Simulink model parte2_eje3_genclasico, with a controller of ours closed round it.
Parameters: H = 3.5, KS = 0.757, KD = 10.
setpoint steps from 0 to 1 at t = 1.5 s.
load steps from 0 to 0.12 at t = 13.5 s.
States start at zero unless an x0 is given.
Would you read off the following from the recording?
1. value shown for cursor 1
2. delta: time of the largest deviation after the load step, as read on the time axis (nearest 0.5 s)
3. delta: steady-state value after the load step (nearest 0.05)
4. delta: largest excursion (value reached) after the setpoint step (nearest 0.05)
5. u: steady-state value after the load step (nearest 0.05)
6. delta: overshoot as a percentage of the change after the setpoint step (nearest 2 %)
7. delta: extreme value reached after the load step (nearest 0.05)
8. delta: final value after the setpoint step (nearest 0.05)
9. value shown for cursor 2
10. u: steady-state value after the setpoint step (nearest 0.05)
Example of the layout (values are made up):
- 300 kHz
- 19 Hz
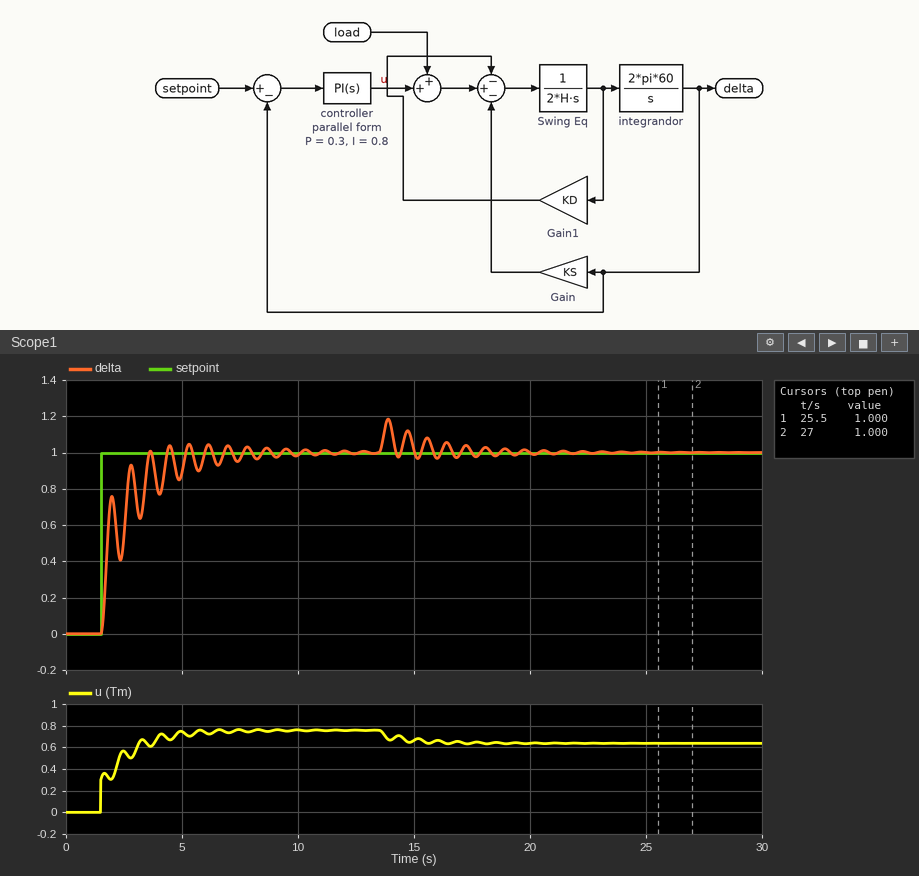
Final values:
- 1.000
- 14.0 s
- 1.00
- 1.05
- 0.65
- 4 %
- 1.20
- 1.00
- 1.000
- 0.75
